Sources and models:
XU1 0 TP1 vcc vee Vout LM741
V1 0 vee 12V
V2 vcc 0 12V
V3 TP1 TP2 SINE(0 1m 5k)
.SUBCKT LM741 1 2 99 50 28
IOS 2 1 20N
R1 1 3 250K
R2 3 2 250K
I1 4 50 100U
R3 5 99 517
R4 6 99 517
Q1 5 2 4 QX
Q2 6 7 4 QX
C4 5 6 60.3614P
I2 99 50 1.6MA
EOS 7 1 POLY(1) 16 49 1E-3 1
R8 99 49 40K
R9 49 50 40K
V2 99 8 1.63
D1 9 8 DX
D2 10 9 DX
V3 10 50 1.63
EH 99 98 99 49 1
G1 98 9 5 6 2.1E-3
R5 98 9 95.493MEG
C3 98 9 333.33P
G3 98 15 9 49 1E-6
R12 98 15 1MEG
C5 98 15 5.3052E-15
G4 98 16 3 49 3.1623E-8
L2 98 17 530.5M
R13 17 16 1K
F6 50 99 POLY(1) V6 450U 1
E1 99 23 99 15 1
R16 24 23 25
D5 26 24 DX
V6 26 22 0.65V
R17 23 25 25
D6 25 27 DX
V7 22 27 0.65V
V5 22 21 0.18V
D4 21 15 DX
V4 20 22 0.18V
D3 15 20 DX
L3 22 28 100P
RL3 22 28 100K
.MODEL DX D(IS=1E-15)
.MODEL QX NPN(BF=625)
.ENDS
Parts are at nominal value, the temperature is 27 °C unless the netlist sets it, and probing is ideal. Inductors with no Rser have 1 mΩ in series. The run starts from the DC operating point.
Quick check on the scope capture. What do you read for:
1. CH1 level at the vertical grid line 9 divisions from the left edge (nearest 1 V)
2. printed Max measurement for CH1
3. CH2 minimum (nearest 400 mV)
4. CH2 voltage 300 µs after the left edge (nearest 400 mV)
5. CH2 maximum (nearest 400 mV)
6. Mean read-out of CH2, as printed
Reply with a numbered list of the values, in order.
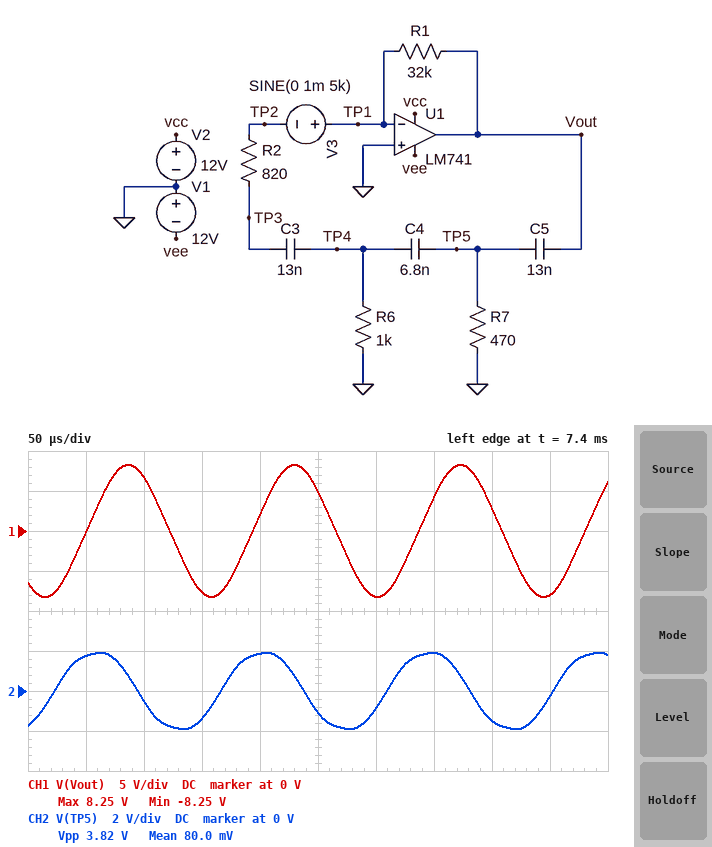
1. -8 V
2. 8.25 V
3. -2.0 V
4. -800 mV
5. 2.0 V
6. 80.0 mV
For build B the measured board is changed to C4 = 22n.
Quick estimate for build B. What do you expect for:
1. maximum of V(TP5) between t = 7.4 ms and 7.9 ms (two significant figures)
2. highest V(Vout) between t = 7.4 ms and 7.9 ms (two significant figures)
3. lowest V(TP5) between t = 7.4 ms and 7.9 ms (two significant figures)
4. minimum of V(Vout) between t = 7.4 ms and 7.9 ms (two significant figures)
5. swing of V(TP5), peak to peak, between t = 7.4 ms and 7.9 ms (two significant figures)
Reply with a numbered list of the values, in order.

1. 1.8 V
2. 11 V
3. -1.8 V
4. -11 V
5. 3.6 V
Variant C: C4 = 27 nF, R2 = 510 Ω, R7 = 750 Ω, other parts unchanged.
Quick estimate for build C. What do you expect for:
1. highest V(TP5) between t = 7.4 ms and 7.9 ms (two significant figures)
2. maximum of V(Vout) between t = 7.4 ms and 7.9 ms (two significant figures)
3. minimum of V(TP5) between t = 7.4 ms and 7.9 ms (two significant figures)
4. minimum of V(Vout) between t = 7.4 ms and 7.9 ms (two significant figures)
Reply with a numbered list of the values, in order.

1. 2.3 V
2. 11 V
3. -2.3 V
4. -11 V
